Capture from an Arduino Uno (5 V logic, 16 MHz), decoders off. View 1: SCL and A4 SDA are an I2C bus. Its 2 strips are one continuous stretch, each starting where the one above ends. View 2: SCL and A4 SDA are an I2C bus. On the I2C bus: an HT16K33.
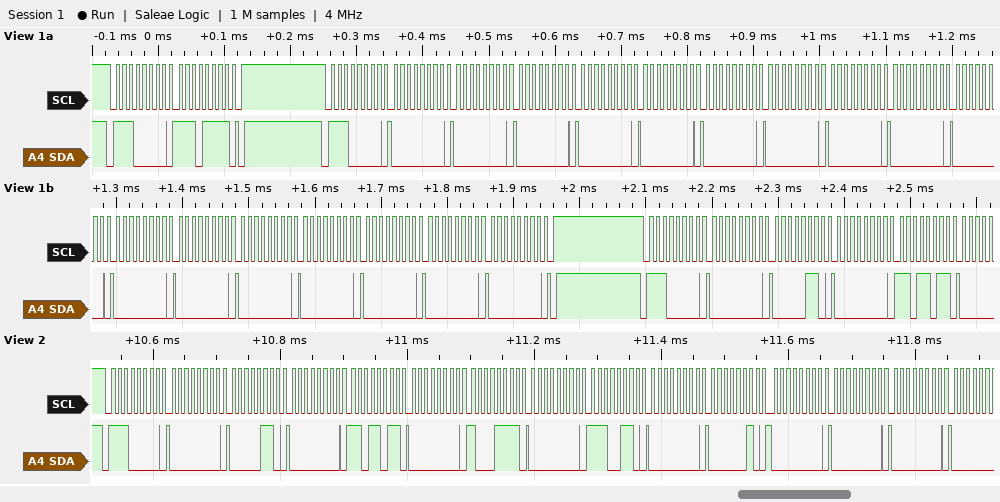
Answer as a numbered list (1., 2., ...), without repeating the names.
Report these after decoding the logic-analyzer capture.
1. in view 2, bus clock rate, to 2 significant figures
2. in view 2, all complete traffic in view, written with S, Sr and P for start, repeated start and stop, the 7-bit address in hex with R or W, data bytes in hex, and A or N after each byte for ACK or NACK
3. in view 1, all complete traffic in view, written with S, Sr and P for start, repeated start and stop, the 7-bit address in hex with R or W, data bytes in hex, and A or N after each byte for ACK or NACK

1. 100 kHz
2. S 70W A 00 A 06 A 00 A DB A 00 A 8F A 00 A E6 A 00 A 02 A 00 A 00 A 00 A
3. S 70W A EF A P S 70W A 00 A 00 A 00 A 00 A 00 A 00 A 00 A 00 A 00 A 00 A 00 A 00 A 00 A 00 A 00 A 00 A 00 A P S 70W A 00 A 06 A 00 A DB A
